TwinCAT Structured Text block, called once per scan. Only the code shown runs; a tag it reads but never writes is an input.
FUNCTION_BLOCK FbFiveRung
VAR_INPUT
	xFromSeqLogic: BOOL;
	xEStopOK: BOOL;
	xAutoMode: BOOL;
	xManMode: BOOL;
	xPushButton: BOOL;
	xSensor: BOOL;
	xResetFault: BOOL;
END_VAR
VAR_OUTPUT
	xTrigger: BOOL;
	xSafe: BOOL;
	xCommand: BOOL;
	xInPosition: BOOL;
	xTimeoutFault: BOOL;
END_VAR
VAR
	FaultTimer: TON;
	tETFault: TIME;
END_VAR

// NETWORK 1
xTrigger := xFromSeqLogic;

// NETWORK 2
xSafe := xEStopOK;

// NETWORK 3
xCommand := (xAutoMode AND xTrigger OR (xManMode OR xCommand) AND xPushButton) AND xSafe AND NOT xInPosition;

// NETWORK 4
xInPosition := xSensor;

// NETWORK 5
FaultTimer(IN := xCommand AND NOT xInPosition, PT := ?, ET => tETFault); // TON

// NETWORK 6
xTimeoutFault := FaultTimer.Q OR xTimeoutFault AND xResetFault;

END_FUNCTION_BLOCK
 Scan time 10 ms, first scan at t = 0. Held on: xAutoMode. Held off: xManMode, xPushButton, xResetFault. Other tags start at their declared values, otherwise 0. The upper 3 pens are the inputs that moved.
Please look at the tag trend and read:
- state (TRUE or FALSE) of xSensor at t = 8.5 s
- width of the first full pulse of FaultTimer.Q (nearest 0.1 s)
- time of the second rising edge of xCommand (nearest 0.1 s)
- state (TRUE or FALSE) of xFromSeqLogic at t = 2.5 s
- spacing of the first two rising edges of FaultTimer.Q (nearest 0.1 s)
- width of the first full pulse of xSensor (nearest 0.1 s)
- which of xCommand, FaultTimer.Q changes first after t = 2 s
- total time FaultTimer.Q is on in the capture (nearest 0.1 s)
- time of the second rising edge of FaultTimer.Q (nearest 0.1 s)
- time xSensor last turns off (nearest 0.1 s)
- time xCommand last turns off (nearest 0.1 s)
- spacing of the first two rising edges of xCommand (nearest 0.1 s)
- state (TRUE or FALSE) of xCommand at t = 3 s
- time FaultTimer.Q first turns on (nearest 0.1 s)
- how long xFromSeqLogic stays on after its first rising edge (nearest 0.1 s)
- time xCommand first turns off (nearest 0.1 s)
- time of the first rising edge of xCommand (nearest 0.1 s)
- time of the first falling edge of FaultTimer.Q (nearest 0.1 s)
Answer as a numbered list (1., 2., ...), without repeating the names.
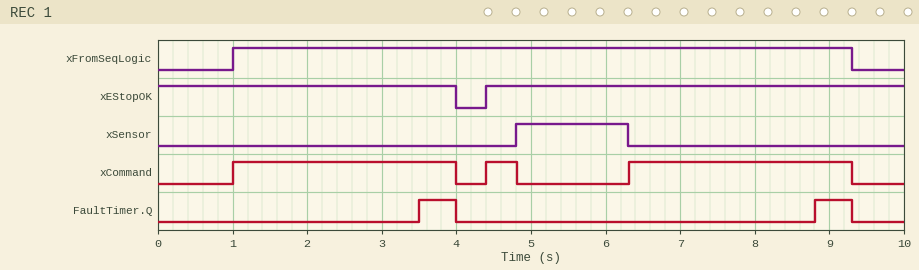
1. FALSE
2. 0.5 s
3. 4.4 s
4. TRUE
5. 5.3 s
6. 1.5 s
7. FaultTimer.Q
8. 1.0 s
9. 8.8 s
10. 6.3 s
11. 9.3 s
12. 3.4 s
13. TRUE
14. 3.5 s
15. 8.3 s
16. 4.0 s
17. 1.0 s
18. 4.0 s
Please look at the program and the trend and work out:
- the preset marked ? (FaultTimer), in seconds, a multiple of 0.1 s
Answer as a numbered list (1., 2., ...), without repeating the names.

1. 2.5 s
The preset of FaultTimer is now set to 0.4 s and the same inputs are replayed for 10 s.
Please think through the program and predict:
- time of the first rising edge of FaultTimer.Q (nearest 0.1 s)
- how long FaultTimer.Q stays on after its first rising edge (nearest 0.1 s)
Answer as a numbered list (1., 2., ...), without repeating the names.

1. 1.4 s
2. 2.6 s
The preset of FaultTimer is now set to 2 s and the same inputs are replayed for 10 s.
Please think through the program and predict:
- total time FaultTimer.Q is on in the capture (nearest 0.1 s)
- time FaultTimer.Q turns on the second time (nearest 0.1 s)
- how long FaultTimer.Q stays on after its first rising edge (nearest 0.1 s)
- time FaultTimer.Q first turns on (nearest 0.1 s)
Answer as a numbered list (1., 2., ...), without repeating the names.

1. 2.0 s
2. 8.3 s
3. 1.0 s
4. 3.0 s
